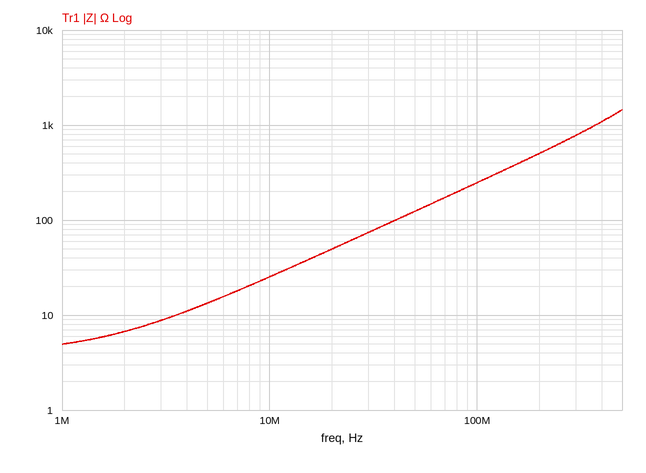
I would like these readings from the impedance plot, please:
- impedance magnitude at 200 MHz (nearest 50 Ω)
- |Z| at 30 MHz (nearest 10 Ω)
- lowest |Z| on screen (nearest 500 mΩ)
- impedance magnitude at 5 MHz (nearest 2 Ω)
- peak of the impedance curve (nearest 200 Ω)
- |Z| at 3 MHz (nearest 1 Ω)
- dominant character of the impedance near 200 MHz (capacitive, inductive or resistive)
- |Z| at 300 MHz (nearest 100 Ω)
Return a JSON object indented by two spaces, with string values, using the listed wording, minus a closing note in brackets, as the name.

{
  "impedance magnitude at 200 MHz": "500 Ω",
  "|Z| at 30 MHz": "70 Ω",
  "lowest |Z| on screen": "5.0 Ω",
  "impedance magnitude at 5 MHz": "14 Ω",
  "peak of the impedance curve": "1.4 kΩ",
  "|Z| at 3 MHz": "9 Ω",
  "dominant character of the impedance near 200 MHz": "inductive",
  "|Z| at 300 MHz": "800 Ω"
}
